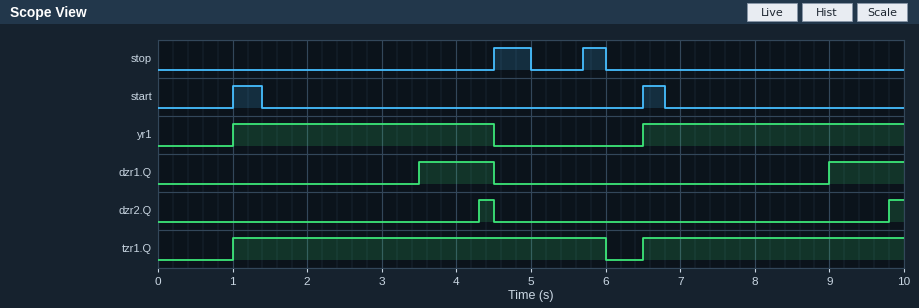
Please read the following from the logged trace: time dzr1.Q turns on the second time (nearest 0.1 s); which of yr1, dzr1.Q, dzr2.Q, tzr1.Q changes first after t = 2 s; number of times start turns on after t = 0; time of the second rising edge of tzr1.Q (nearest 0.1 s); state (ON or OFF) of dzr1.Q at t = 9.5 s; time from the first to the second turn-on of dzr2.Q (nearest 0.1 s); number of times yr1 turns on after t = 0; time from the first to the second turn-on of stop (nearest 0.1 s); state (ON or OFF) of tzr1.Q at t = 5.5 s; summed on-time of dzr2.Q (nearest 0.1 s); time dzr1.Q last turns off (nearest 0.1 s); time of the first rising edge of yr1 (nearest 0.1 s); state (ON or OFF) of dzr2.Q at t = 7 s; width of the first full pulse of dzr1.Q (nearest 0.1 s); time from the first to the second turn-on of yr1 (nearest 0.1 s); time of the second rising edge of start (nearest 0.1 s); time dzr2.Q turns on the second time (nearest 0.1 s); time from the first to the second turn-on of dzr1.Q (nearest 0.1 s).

9.0 s
dzr1.Q
2
6.5 s
ON
5.5 s
2
1.2 s
ON
0.4 s
4.5 s
1.0 s
OFF
1.0 s
5.5 s
6.5 s
9.8 s
5.5 s
